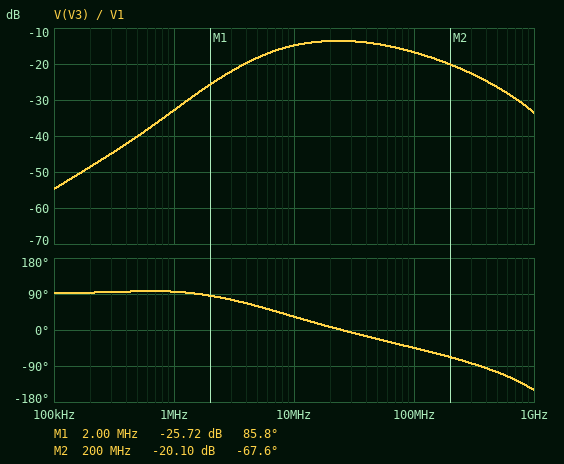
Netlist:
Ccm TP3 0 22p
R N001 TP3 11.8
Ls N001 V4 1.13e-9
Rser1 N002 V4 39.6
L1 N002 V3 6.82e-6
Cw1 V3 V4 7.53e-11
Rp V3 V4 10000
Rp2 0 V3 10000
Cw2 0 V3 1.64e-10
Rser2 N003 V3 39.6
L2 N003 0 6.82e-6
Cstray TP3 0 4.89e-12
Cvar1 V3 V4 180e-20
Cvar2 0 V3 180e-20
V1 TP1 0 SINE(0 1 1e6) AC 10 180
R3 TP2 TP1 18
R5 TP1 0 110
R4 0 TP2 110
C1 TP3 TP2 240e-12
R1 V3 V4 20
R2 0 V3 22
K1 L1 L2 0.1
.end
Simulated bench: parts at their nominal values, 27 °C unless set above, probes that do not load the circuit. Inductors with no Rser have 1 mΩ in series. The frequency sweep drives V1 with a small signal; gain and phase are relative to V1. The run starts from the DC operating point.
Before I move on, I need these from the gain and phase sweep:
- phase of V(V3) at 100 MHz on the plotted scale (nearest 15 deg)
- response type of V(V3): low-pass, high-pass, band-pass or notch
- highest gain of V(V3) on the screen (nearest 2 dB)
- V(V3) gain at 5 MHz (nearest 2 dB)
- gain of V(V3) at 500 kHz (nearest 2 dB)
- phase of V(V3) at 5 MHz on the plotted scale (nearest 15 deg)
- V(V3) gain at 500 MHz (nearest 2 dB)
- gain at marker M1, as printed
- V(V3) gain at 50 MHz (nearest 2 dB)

-45 deg
band-pass
-14 dB
-18 dB
-40 dB
60 deg
-26 dB
-25.72 dB
-14 dB
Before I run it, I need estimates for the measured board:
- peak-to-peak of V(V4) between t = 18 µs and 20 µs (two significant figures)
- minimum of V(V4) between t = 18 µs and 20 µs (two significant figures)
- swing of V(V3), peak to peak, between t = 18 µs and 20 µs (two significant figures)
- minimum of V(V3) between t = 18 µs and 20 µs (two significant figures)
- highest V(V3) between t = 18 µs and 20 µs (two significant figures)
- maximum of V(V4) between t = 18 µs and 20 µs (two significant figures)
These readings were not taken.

88 mV
-44 mV
46 mV
-23 mV
23 mV
44 mV
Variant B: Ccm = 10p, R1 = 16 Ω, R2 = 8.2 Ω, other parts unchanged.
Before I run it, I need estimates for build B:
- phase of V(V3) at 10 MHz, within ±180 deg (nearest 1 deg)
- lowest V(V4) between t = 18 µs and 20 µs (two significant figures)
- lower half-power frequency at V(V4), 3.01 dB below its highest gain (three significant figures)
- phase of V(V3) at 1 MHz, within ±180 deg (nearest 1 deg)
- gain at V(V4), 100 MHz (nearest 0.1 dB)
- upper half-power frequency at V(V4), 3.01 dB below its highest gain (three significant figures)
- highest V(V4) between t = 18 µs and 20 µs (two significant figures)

47 deg
-27 mV
10.8 MHz
91 deg
-9.3 dB
262 MHz
27 mV
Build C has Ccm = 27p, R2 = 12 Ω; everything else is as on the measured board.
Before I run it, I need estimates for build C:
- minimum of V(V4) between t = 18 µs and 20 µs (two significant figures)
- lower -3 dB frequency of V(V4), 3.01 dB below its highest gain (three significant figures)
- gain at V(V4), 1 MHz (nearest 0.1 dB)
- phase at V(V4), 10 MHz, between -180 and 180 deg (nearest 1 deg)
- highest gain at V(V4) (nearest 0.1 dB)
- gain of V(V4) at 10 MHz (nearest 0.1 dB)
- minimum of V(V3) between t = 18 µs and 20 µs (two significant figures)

-35 mV
8.77 MHz
-29.2 dB
42 deg
-8.3 dB
-10.7 dB
-14 mV
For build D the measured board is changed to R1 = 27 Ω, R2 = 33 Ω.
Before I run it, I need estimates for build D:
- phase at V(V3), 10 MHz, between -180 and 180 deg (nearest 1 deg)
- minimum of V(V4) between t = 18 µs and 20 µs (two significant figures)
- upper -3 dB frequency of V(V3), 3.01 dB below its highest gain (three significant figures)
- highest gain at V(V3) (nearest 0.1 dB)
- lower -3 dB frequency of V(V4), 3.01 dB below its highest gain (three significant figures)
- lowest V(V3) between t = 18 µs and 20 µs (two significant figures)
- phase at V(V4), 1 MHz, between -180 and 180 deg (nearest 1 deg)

24 deg
-58 mV
73.1 MHz
-12.4 dB
5.44 MHz
-31 mV
98 deg
